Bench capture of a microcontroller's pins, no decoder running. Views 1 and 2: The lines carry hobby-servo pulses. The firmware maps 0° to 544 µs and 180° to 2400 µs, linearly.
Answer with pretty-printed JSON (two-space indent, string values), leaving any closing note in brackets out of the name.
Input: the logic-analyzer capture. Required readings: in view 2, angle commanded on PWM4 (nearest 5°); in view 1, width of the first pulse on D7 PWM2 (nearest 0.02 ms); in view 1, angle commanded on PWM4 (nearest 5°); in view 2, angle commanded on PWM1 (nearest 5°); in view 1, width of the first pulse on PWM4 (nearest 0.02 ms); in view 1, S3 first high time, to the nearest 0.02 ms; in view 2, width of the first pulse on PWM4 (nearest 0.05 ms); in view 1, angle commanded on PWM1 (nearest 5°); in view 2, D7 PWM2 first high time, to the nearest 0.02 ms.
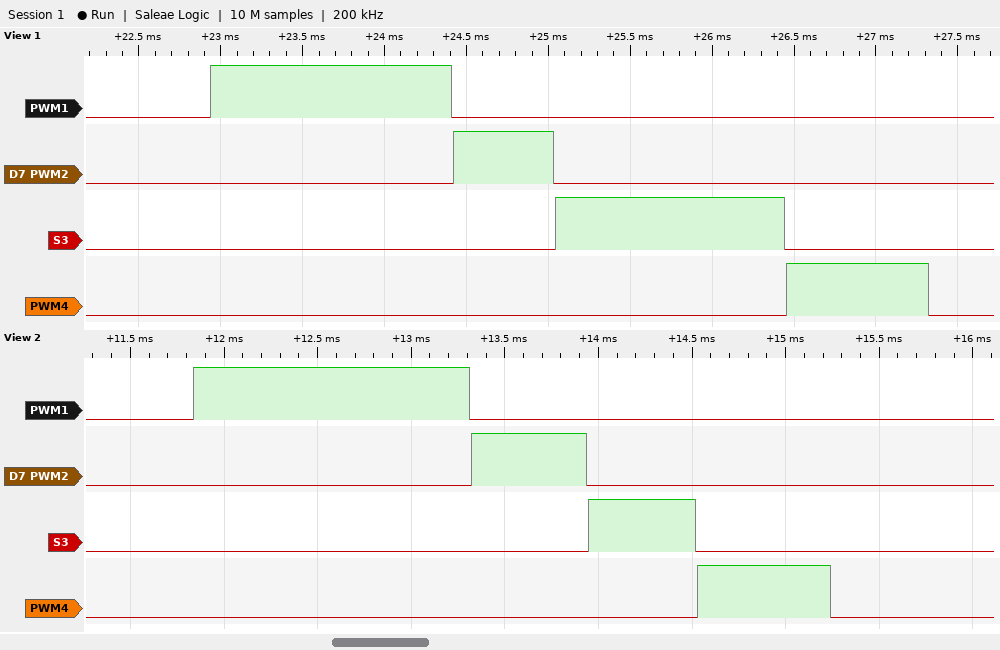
{
  "in view 2, angle commanded on PWM4": "15°",
  "in view 1, width of the first pulse on D7 PWM2": "0.62 ms",
  "in view 1, angle commanded on PWM4": "30°",
  "in view 2, angle commanded on PWM1": "90°",
  "in view 1, width of the first pulse on PWM4": "0.86 ms",
  "in view 1, S3 first high time, to the nearest 0.02 ms": "1.40 ms",
  "in view 2, width of the first pulse on PWM4": "0.70 ms",
  "in view 1, angle commanded on PWM1": "90°",
  "in view 2, D7 PWM2 first high time, to the nearest 0.02 ms": "0.62 ms"
}
